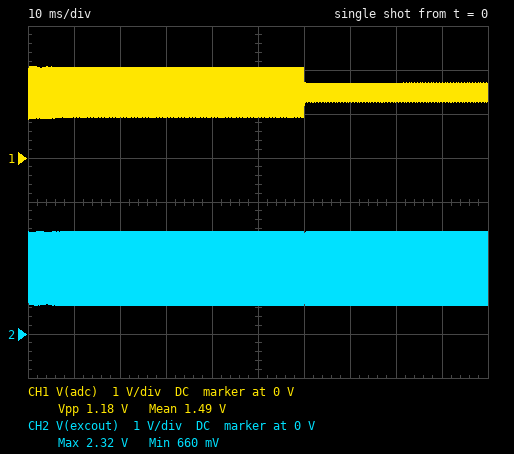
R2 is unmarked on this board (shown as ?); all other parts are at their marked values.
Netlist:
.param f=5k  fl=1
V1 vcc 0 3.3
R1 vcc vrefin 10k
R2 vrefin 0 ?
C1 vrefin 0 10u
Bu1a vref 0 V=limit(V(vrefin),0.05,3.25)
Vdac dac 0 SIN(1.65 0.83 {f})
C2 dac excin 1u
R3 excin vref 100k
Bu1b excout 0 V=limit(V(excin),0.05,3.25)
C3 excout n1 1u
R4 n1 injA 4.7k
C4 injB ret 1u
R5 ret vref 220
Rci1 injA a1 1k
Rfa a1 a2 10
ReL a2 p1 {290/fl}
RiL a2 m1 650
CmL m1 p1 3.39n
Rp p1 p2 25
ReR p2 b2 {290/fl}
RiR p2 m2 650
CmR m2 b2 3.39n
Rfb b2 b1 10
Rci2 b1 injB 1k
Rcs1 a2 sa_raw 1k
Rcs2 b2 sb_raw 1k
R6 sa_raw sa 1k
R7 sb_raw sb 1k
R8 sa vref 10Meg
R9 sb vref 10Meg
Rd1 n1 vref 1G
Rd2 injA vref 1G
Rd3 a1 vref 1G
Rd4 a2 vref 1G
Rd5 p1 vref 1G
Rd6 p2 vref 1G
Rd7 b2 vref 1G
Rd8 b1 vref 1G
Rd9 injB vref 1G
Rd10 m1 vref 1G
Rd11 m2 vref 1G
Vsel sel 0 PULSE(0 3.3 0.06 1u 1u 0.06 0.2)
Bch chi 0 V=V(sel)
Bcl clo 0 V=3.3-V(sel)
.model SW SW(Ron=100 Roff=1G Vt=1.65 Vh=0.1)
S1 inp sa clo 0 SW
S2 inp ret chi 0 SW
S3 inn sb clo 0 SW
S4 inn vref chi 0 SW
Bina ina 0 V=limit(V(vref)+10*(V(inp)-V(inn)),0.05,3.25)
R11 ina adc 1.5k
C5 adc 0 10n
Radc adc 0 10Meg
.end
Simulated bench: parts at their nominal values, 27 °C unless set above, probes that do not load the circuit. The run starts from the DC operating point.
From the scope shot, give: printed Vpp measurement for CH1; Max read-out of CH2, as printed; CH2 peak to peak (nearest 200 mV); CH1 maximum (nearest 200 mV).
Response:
1.18 V
2.32 V
1.6 V
2.0 V
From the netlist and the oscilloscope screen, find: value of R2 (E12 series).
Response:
8.2 kΩ
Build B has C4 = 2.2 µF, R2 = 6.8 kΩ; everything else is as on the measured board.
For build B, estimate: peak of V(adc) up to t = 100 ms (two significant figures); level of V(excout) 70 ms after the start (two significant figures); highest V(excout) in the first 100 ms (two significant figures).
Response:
1.9 V
1.3 V
2.2 V
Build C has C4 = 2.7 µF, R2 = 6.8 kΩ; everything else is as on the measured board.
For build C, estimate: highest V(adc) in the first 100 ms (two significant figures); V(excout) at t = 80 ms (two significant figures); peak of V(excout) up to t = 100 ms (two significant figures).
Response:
1.9 V
1.3 V
2.2 V
